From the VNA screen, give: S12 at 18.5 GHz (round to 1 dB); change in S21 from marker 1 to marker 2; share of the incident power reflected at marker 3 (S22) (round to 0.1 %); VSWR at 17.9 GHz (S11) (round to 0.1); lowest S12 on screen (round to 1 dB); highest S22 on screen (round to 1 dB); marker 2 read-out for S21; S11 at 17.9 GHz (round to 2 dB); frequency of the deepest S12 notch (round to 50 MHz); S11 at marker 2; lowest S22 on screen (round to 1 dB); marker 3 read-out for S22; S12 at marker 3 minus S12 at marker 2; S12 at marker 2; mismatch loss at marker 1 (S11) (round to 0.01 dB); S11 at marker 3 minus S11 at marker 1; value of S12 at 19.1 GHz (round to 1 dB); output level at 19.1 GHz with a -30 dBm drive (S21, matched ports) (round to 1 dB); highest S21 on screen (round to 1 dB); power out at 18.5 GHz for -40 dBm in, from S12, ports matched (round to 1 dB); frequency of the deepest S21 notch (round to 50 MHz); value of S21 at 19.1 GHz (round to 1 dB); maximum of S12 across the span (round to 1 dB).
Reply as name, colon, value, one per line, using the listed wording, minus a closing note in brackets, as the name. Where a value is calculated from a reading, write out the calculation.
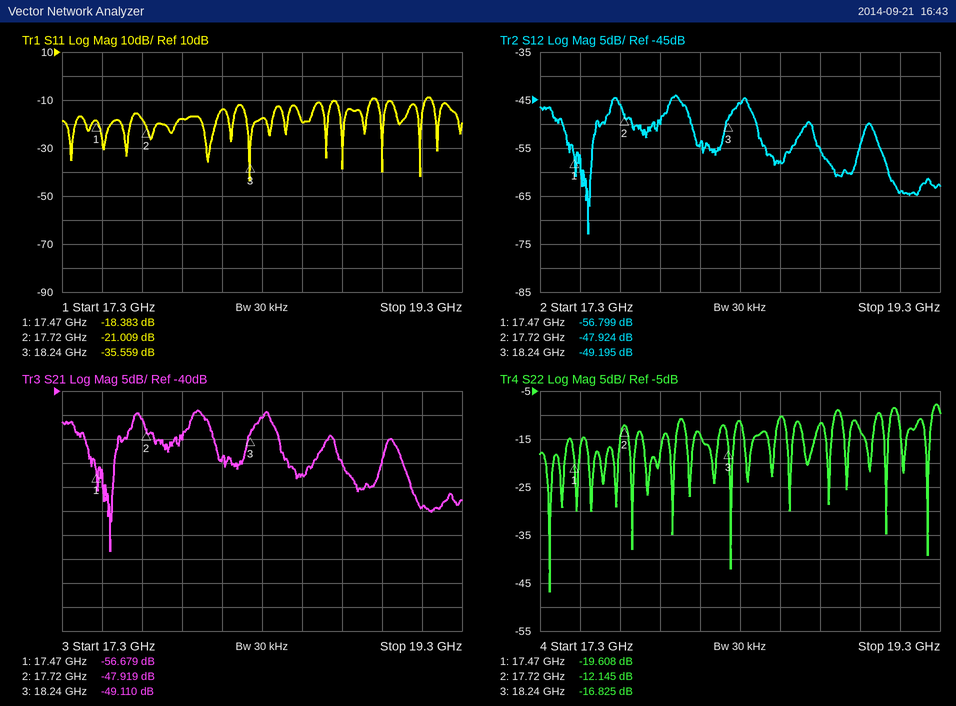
S12 at 18.5 GHz: -58 dB
change in S21 from marker 1 to marker 2: -47.919 − (-56.679) = 8.760 dB
share of the incident power reflected at marker 3 (S22): 10^(-16.825/10) ≈ 2.1 %
VSWR at 17.9 GHz (S11): |Γ| = 10^(-18/20) = 0.1259; VSWR = (1 + 0.1259)/(1 − 0.1259) ≈ 1.3
lowest S12 on screen: -73 dB
highest S22 on screen: -8 dB
marker 2 read-out for S21: -47.919 dB
S11 at 17.9 GHz: -18 dB
frequency of the deepest S12 notch: 17.55 GHz
S11 at marker 2: -21.009 dB
lowest S22 on screen: -47 dB
marker 3 read-out for S22: -16.825 dB
S12 at marker 3 minus S12 at marker 2: -49.195 − (-47.924) = -1.271 dB
S12 at marker 2: -47.924 dB
mismatch loss at marker 1 (S11): −10 log10(1 − 10^(-18.383/10)) ≈ 0.06 dB
S11 at marker 3 minus S11 at marker 1: -35.559 − (-18.383) = -17.176 dB
value of S12 at 19.1 GHz: -64 dB
output level at 19.1 GHz with a -30 dBm drive (S21, matched ports): -30 dBm + (-64 dB) = -94 dBm
highest S21 on screen: -44 dB
power out at 18.5 GHz for -40 dBm in, from S12, ports matched: -40 dBm + (-58 dB) = -98 dBm
frequency of the deepest S21 notch: 17.55 GHz
value of S21 at 19.1 GHz: -64 dB
maximum of S12 across the span: -44 dB
